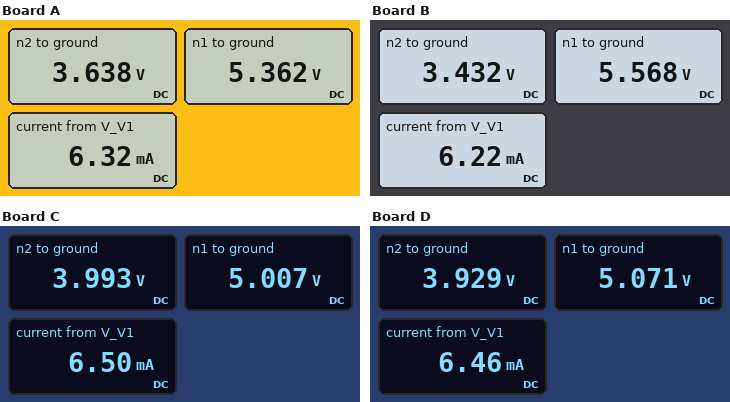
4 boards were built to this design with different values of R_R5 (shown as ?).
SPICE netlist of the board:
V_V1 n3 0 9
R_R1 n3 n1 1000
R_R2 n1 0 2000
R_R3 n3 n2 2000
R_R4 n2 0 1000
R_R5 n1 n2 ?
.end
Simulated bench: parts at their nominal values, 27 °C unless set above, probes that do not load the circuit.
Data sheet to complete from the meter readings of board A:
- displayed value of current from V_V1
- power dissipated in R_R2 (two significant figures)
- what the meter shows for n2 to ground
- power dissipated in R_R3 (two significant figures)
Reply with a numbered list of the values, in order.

1. 6.32 mA
2. 14 mW
3. 3.638 V
4. 14 mW
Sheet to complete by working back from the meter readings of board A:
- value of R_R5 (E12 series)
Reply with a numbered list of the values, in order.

1. 1.8 kΩ
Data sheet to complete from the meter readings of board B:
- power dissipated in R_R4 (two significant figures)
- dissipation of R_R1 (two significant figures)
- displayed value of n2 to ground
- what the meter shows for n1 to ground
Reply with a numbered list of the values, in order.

1. 12 mW
2. 12 mW
3. 3.432 V
4. 5.568 V
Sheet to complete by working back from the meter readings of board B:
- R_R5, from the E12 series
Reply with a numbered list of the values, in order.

1. 3.3 kΩ
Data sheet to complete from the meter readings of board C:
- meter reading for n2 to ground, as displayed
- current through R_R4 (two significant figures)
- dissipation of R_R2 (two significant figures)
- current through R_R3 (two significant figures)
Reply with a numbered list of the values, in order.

1. 3.993 V
2. 4.0 mA
3. 13 mW
4. 2.5 mA
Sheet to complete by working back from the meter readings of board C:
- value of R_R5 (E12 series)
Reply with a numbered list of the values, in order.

1. 680 Ω
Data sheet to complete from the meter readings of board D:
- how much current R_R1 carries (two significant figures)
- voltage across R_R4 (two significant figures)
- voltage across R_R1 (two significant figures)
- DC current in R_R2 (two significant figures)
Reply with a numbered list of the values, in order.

1. 3.9 mA
2. 3.9 V
3. 3.9 V
4. 2.5 mA
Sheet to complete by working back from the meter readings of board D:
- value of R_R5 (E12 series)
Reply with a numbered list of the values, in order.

1. 820 Ω
